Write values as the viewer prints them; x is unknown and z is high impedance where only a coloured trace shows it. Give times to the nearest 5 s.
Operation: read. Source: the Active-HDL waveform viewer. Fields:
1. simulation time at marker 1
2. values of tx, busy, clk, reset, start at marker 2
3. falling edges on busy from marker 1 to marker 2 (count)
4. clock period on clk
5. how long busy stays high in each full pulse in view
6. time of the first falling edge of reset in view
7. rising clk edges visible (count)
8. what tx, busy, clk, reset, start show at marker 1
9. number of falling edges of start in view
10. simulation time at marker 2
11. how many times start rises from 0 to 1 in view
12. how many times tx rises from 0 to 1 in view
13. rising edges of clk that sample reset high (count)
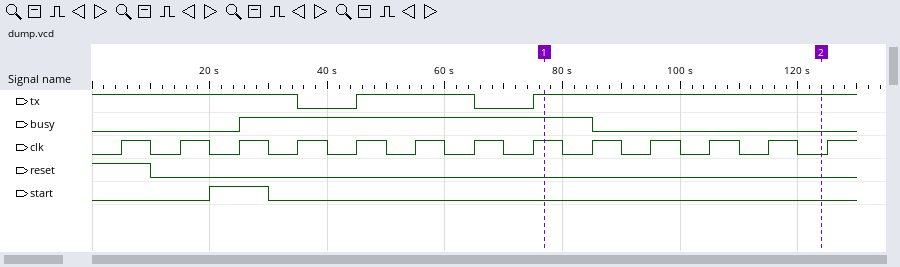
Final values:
75 s
tx=1, busy=0, clk=0, reset=0, start=0
1
10 s
60 s
10 s
13
tx=1, busy=1, clk=1, reset=0, start=0
1
125 s
1
2
1
